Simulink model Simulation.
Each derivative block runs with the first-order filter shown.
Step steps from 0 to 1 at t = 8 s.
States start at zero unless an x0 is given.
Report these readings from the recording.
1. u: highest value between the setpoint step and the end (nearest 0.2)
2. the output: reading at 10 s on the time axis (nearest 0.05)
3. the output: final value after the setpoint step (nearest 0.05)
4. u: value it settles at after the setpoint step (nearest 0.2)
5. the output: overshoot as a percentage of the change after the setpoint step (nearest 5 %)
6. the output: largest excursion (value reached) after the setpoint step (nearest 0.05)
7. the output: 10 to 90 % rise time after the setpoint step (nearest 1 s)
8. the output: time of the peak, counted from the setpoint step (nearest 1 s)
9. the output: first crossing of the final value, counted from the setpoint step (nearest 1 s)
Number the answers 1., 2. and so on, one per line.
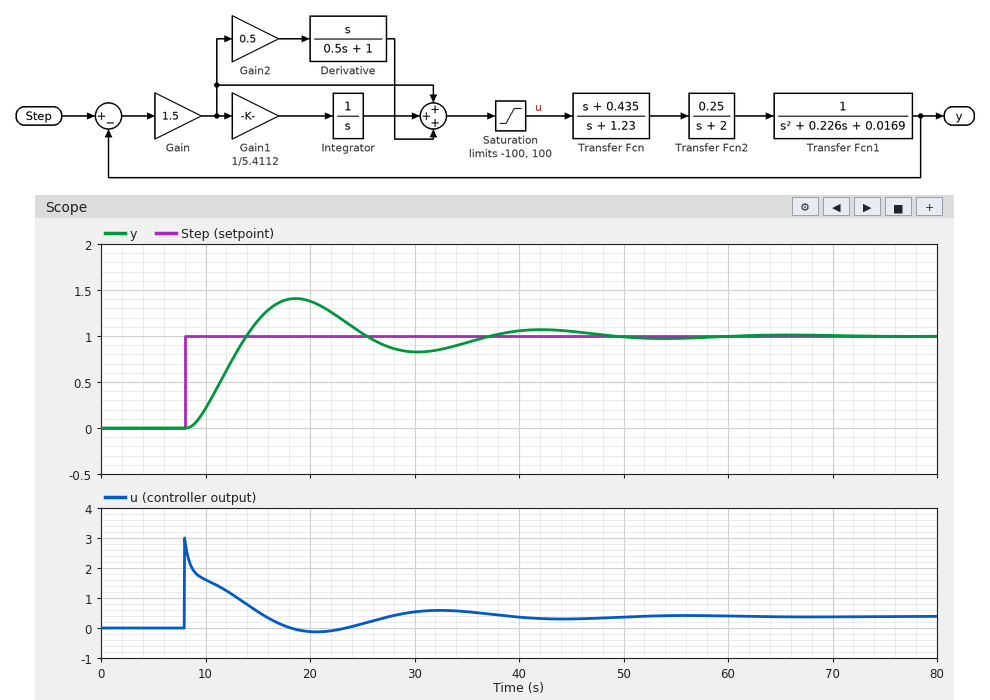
1. 3.0
2. 0.20
3. 1.00
4. 0.4
5. 40 %
6. 1.40
7. 4 s
8. 11 s
9. 6 s
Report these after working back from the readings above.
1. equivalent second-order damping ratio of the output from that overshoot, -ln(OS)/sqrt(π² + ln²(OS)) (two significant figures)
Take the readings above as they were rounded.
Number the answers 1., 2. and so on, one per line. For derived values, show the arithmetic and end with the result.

1. ln(0.4) = -0.916; 0.916 / sqrt(9.870 + 0.840) = 0.28
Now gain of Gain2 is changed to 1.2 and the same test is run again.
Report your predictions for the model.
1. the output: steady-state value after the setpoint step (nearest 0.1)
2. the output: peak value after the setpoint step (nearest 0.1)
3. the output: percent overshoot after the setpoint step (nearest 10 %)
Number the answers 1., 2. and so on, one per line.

1. 1.0
2. 1.3
3. 30 %
